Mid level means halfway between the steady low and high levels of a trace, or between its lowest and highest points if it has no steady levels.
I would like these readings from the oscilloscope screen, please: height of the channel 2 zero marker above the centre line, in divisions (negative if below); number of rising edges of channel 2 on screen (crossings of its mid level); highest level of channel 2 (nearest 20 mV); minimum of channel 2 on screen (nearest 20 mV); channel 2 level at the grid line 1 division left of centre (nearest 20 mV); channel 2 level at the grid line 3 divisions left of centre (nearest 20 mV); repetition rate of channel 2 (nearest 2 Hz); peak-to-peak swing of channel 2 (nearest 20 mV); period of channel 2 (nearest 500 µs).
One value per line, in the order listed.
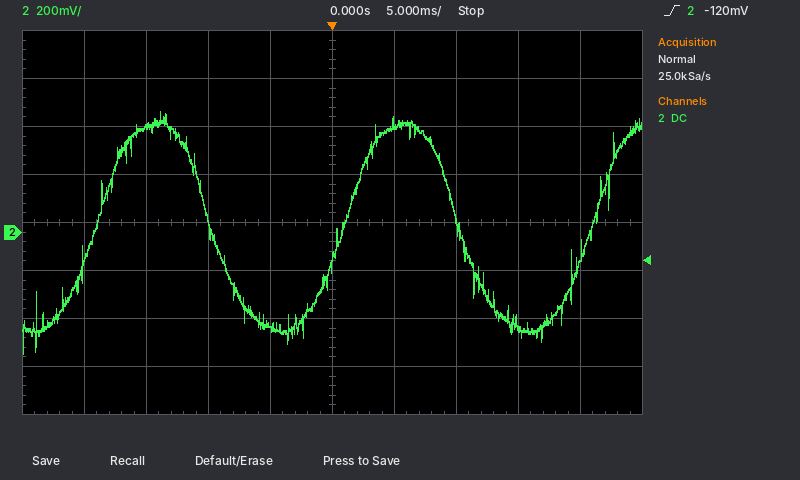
-0.2 div
3
500 mV
-500 mV
-400 mV
440 mV
50 Hz
1.00 V
20.0 ms
